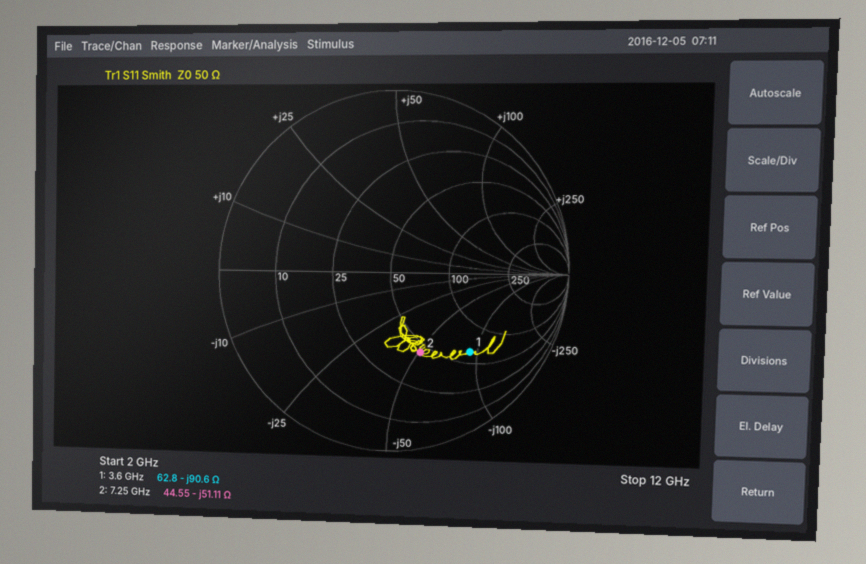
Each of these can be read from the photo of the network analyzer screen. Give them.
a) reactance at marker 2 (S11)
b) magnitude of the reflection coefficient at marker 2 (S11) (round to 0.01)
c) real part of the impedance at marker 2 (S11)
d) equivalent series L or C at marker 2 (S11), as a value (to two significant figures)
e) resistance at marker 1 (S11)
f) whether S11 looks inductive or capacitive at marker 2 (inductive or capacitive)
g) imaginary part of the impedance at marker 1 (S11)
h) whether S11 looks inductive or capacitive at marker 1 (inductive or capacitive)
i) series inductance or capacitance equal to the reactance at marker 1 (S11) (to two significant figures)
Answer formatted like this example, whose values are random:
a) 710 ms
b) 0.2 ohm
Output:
a) -51.11 Ω
b) 0.48
c) 44.55 Ω
d) 430 fF
e) 62.8 Ω
f) capacitive
g) -90.6 Ω
h) capacitive
i) 490 fF
